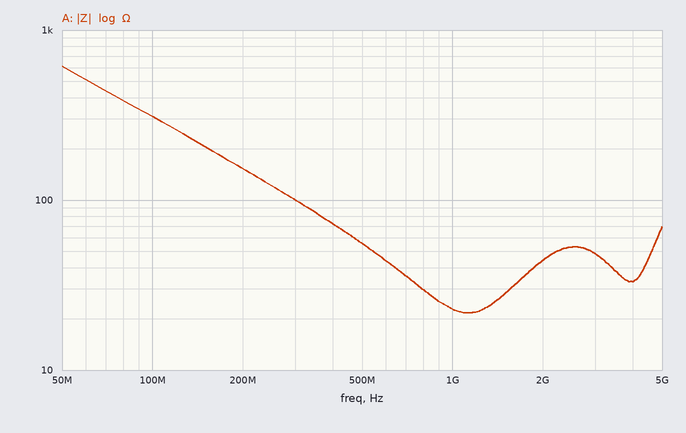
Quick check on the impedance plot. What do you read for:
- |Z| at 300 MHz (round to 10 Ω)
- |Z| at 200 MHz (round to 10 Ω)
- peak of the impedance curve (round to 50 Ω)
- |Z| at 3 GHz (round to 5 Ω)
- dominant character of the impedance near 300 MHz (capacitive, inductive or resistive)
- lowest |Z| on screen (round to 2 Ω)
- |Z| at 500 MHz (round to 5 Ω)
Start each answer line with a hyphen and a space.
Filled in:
- 100 Ω
- 150 Ω
- 600 Ω
- 50 Ω
- capacitive
- 22 Ω
- 55 Ω
